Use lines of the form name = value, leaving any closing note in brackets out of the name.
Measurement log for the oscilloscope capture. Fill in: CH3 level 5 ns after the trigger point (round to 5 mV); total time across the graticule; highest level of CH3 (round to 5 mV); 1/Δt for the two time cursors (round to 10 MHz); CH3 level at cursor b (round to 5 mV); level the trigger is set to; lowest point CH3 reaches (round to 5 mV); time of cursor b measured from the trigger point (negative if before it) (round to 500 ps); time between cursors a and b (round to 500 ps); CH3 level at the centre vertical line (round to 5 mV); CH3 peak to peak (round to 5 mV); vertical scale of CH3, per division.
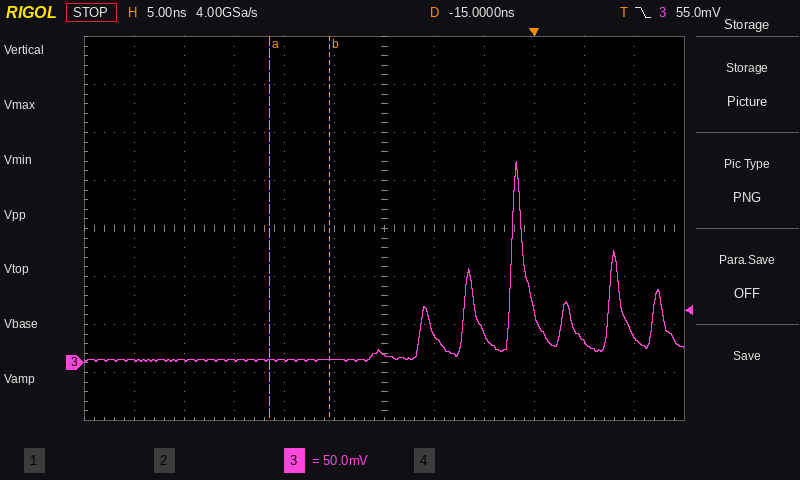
CH3 level 5 ns after the trigger point = 20 mV
total time across the graticule = 60 ns
highest level of CH3 = 210 mV
1/Δt for the two time cursors = 170 MHz
CH3 level at cursor b = 5 mV
level the trigger is set to = 55.0 mV
lowest point CH3 reaches = 0 mV
time of cursor b measured from the trigger point (negative if before it) = -20.5 ns
time between cursors a and b = 6.0 ns
CH3 level at the centre vertical line = 10 mV
CH3 peak to peak = 210 mV
vertical scale of CH3, per division = 50 mV
